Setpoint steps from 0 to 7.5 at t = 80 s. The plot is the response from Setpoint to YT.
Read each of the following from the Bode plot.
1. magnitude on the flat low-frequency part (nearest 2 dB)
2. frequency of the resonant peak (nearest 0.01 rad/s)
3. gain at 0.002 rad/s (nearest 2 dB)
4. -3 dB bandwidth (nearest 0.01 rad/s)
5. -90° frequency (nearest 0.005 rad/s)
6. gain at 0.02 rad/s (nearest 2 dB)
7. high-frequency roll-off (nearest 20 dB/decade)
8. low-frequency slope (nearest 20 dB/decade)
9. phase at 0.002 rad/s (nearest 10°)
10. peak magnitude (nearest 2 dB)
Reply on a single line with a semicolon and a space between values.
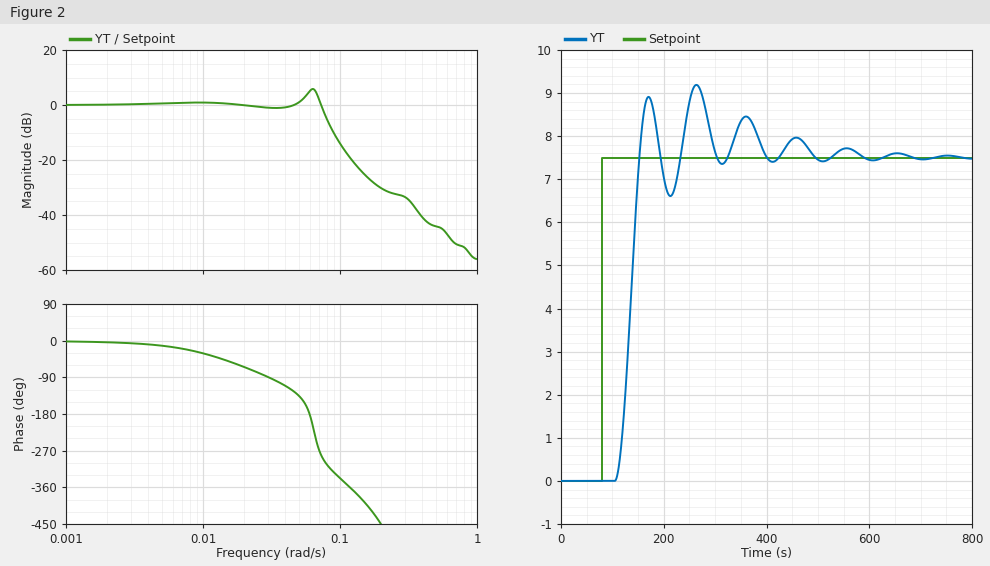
0 dB; 0.06 rad/s; 0 dB; 0.08 rad/s; 0.030 rad/s; 0 dB; -40 dB/decade; 0 dB/decade; 0°; 6 dB
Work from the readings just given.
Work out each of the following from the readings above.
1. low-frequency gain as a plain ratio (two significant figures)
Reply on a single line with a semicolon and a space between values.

1.0
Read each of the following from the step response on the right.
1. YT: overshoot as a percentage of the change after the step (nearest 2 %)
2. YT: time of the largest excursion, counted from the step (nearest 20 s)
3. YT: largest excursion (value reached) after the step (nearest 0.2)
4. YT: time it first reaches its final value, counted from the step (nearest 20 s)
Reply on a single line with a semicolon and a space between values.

22 %; 180 s; 9.2; 80 s
